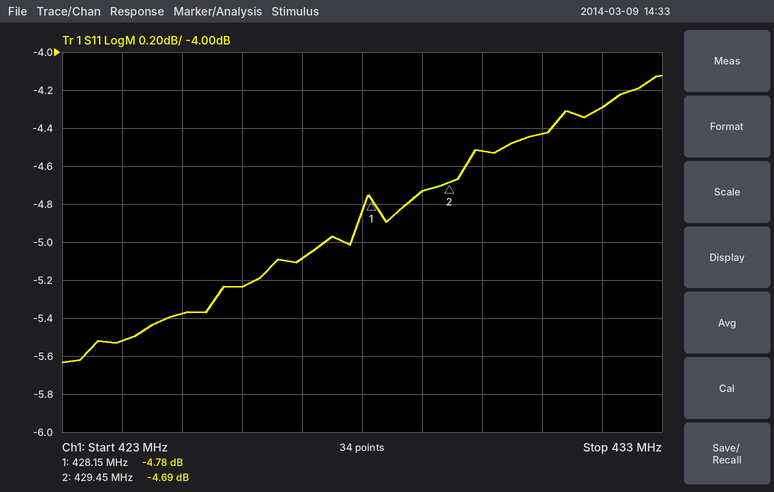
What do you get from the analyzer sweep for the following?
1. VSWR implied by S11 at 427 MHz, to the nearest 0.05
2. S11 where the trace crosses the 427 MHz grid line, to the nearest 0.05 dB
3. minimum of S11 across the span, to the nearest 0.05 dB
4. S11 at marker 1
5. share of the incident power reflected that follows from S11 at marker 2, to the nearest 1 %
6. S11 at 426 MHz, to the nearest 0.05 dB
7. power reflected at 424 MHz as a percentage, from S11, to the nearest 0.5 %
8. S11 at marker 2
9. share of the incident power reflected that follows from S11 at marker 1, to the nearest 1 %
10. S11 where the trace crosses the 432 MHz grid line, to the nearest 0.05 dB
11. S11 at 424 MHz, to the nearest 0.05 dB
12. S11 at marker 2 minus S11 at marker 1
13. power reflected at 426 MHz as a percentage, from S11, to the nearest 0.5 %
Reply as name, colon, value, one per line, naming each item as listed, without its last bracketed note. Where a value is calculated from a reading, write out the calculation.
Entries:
VSWR implied by S11 at 427 MHz, to the nearest 0.05: |Γ| = 10^(-5.1/20) = 0.5559; VSWR = (1 + 0.5559)/(1 − 0.5559) ≈ 3.50
S11 where the trace crosses the 427 MHz grid line, to the nearest 0.05 dB: -5.10 dB
minimum of S11 across the span, to the nearest 0.05 dB: -5.65 dB
S11 at marker 1: -4.78 dB
share of the incident power reflected that follows from S11 at marker 2, to the nearest 1 %: 10^(-4.69/10) ≈ 34 %
S11 at 426 MHz, to the nearest 0.05 dB: -5.25 dB
power reflected at 424 MHz as a percentage, from S11, to the nearest 0.5 %: 10^(-5.5/10) ≈ 28.2 %, so 28.0 % to the nearest 0.5 %
S11 at marker 2: -4.69 dB
share of the incident power reflected that follows from S11 at marker 1, to the nearest 1 %: 10^(-4.78/10) ≈ 33 %
S11 where the trace crosses the 432 MHz grid line, to the nearest 0.05 dB: -4.30 dB
S11 at 424 MHz, to the nearest 0.05 dB: -5.50 dB
S11 at marker 2 minus S11 at marker 1: -4.69 − (-4.78) = 0.09 dB
power reflected at 426 MHz as a percentage, from S11, to the nearest 0.5 %: 10^(-5.25/10) ≈ 29.9 %, so 30.0 % to the nearest 0.5 %
